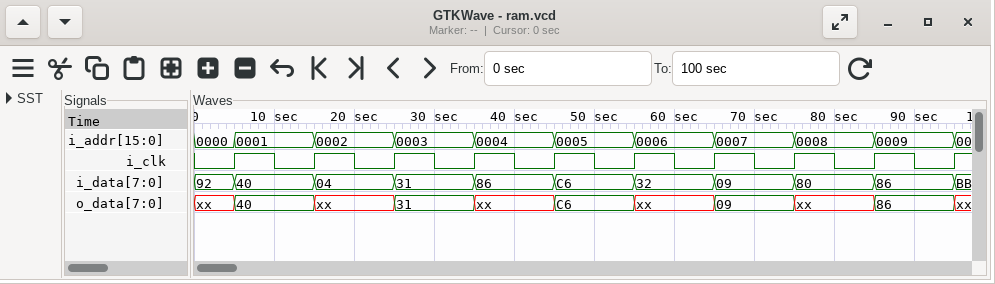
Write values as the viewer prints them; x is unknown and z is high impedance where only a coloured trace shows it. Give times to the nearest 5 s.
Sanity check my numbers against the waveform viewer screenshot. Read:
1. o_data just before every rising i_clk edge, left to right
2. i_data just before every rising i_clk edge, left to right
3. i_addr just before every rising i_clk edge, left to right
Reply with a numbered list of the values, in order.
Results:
1. xx, 40, xx, 31, xx, C6, xx, 09, xx, 86
2. 92, 40, 04, 31, 86, C6, 32, 09, 80, 86
3. 0000, 0001, 0002, 0003, 0004, 0005, 0006, 0007, 0008, 0009
